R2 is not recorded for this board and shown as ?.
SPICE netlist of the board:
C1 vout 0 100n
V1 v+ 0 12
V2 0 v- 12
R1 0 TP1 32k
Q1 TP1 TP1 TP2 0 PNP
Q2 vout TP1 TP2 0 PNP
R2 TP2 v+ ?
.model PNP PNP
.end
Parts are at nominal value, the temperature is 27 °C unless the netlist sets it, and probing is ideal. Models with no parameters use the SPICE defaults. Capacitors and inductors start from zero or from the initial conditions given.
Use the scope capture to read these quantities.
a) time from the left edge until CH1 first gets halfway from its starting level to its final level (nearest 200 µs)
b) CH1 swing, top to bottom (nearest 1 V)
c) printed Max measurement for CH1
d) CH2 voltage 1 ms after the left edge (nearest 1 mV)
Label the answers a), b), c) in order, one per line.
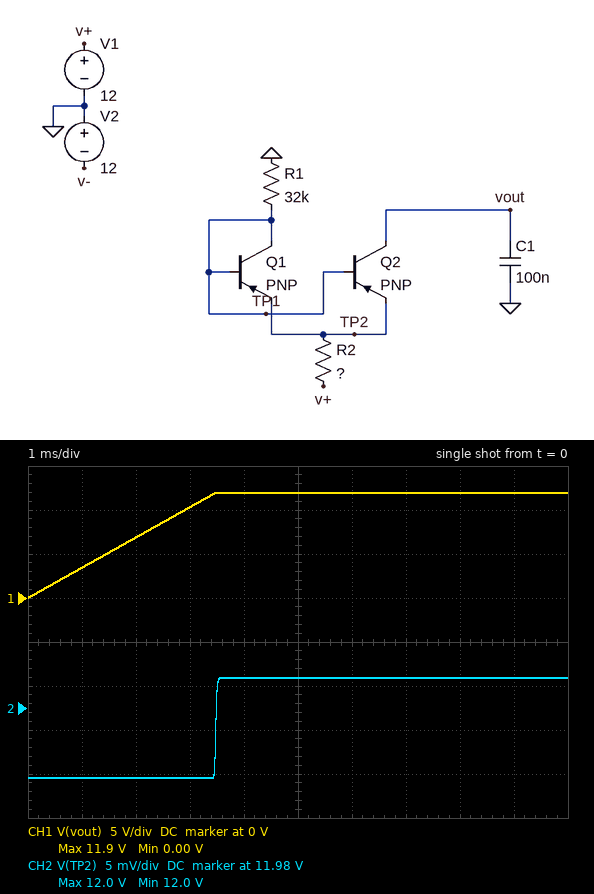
a) 1.8 ms
b) 12 V
c) 11.9 V
d) 11.977 V
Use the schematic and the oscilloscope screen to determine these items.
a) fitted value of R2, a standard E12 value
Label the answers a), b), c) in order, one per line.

a) 33 Ω
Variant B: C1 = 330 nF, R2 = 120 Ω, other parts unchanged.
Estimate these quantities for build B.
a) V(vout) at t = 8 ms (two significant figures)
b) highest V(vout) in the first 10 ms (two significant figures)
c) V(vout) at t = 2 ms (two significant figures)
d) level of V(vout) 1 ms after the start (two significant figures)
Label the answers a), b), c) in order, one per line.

a) 8.3 V
b) 10 V
c) 2.1 V
d) 1.0 V
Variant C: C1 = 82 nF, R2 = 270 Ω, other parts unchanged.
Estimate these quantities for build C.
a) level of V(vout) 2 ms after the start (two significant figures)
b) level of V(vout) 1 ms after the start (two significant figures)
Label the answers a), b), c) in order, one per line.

a) 8.3 V
b) 4.1 V
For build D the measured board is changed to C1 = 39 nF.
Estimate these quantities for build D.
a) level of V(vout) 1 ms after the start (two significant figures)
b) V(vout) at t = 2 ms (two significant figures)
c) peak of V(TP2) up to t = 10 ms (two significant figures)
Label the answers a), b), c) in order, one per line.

a) 8.8 V
b) 12 V
c) 12 V
